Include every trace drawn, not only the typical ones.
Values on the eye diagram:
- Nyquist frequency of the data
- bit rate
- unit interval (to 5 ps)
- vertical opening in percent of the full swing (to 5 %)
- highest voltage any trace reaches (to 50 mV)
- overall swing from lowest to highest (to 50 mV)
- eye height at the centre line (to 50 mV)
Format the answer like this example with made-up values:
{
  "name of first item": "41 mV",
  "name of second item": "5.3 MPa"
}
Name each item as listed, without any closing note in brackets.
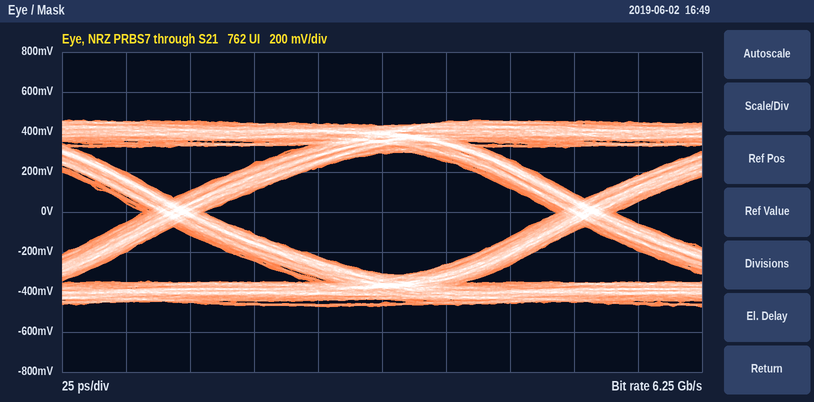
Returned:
{
  "Nyquist frequency of the data": "3.125 GHz",
  "bit rate": "6.25 Gb/s",
  "unit interval": "160 ps",
  "vertical opening in percent of the full swing": "65 %",
  "highest voltage any trace reaches": "450 mV",
  "overall swing from lowest to highest": "950 mV",
  "eye height at the centre line": "600 mV"
}
